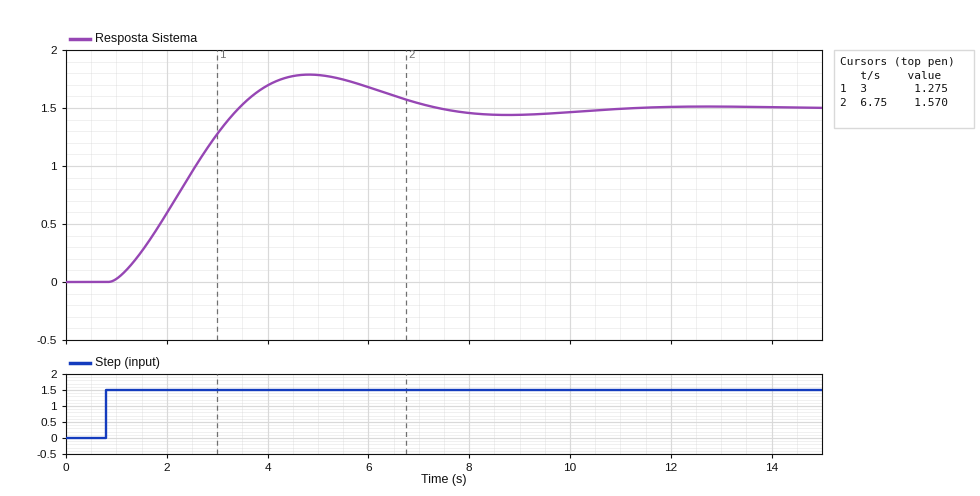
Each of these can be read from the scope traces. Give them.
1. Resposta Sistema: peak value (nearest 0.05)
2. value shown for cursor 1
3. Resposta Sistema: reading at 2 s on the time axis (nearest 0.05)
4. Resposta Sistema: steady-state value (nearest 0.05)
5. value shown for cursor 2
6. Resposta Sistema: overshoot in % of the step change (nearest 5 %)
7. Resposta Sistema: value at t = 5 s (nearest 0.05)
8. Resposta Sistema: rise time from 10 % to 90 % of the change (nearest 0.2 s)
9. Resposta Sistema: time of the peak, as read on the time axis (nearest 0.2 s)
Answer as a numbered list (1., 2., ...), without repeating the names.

1. 1.80
2. 1.275
3. 0.60
4. 1.50
5. 1.570
6. 20 %
7. 1.80
8. 1.8 s
9. 4.8 s
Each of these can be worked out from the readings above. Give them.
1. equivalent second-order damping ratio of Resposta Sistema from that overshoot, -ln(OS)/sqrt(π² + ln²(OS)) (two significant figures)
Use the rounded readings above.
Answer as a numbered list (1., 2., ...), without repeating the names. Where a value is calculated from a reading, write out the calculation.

1. ln(0.2) = -1.609; 1.609 / sqrt(9.870 + 2.590) = 0.46
